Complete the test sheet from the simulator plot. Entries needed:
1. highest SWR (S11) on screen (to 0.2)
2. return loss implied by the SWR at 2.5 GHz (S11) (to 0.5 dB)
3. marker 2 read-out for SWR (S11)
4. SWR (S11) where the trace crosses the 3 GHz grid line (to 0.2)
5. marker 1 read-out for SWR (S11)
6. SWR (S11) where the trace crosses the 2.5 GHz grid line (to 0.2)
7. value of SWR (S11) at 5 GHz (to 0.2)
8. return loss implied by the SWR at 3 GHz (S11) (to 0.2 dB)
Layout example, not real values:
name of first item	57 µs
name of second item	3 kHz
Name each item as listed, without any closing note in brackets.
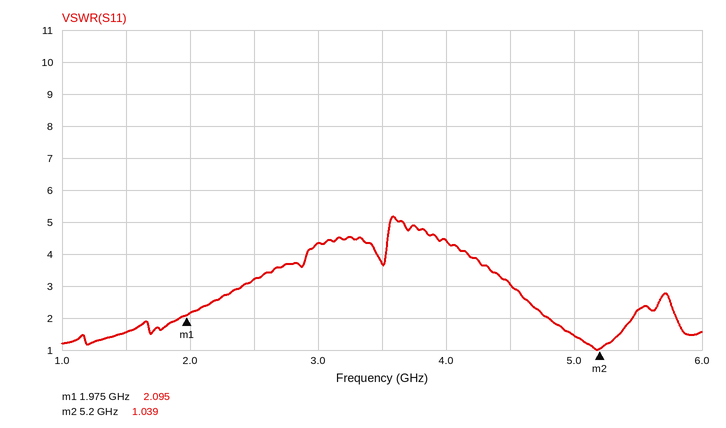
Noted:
highest SWR (S11) on screen	5.2
return loss implied by the SWR at 2.5 GHz (S11)	5.5 dB
marker 2 read-out for SWR	1.039
SWR (S11) where the trace crosses the 3 GHz grid line	4.4
marker 1 read-out for SWR	2.095
SWR (S11) where the trace crosses the 2.5 GHz grid line	3.2
value of SWR (S11) at 5 GHz	1.4
return loss implied by the SWR at 3 GHz (S11)	4.0 dB
